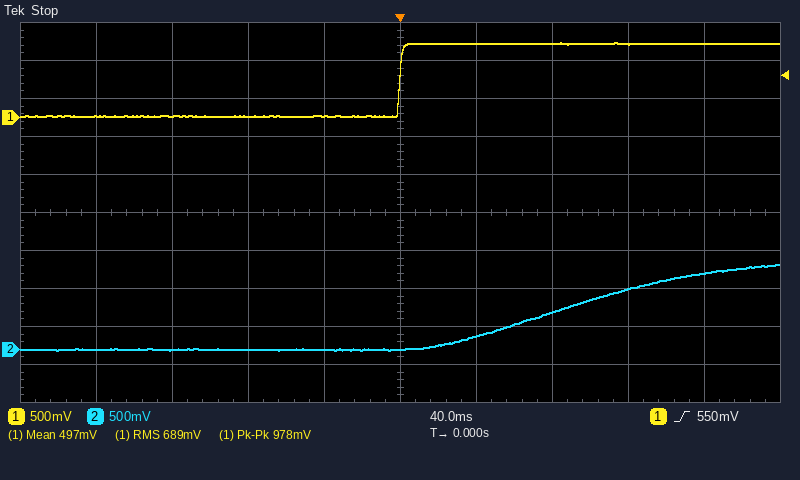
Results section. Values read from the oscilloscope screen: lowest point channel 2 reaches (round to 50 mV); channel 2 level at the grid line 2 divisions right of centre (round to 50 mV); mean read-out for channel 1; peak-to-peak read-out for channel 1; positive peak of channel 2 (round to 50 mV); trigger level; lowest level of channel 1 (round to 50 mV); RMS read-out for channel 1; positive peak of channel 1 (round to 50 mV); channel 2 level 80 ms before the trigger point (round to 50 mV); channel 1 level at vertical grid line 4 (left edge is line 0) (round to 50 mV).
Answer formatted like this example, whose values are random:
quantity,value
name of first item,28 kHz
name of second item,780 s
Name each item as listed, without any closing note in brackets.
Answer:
quantity,value
lowest point channel 2 reaches,0 mV
channel 2 level at the grid line 2 divisions right of centre,500 mV
mean read-out for channel 1,497 mV
peak-to-peak read-out for channel 1,978 mV
positive peak of channel 2,1.10 V
trigger level,550 mV
lowest level of channel 1,0 mV
RMS read-out for channel 1,689 mV
positive peak of channel 1,1.00 V
channel 2 level 80 ms before the trigger point,0 mV
channel 1 level at vertical grid line 4 (left edge is line 0),0 mV
